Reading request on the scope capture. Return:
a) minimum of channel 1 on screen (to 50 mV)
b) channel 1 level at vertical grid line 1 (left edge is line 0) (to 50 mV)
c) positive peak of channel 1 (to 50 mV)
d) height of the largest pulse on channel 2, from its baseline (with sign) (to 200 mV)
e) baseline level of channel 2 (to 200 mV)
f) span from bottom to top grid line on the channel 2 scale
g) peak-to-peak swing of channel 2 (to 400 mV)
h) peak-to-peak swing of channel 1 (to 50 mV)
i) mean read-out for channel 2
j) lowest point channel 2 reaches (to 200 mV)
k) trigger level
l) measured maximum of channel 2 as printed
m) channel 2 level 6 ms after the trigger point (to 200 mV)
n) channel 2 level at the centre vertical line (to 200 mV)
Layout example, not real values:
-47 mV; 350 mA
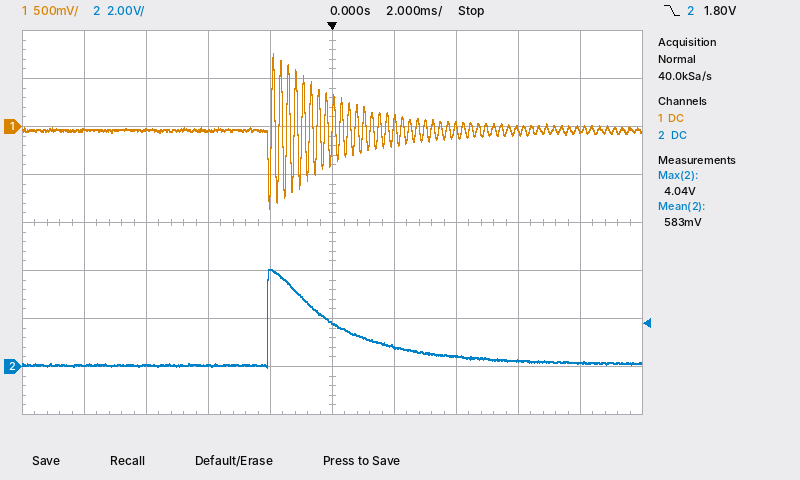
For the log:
-850 mV; -50 mV; 750 mV; +4.0 V; 0.0 V; 16 V; 4.0 V; 1.60 V; 583 mV; 0.0 V; 1.80 V; 4.04 V; 200 mV; 1.8 V
